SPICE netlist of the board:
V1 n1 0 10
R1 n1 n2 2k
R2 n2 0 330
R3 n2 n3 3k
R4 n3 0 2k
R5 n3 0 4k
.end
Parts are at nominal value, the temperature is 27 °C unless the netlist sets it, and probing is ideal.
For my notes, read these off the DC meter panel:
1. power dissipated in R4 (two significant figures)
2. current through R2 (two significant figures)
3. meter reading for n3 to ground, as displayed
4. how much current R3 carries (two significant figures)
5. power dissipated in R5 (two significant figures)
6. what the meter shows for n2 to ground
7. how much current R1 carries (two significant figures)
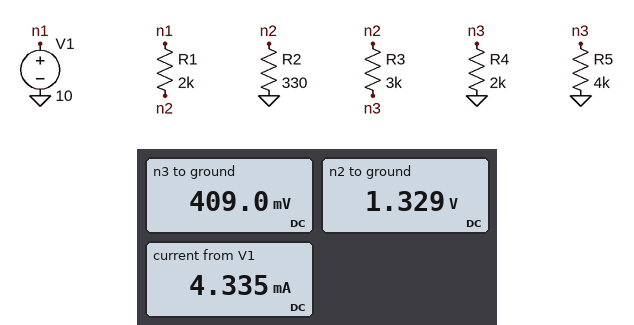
84 µW
4.0 mA
409.0 mV
310 µA
42 µW
1.329 V
4.3 mA
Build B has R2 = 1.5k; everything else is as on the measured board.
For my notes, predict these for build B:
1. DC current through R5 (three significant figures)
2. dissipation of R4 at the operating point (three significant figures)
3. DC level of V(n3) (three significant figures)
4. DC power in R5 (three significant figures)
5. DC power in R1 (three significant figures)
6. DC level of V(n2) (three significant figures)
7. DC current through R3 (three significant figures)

275 µA
606 µW
1.10 V
303 µW
20.6 mW
3.58 V
826 µA
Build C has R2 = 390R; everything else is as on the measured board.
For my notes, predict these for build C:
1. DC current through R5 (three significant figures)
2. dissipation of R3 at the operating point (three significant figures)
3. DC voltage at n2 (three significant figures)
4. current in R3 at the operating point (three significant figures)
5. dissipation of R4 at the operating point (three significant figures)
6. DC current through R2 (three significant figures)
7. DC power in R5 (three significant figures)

117 µA
368 µW
1.52 V
350 µA
109 µW
3.89 mA
54.5 µW
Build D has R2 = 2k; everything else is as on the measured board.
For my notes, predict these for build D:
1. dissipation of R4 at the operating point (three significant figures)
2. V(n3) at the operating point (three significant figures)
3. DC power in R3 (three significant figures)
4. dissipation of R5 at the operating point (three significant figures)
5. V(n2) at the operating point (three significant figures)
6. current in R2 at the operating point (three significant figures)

781 µW
1.25 V
2.64 mW
391 µW
4.06 V
2.03 mA
